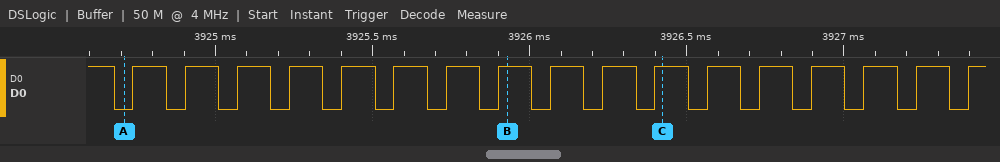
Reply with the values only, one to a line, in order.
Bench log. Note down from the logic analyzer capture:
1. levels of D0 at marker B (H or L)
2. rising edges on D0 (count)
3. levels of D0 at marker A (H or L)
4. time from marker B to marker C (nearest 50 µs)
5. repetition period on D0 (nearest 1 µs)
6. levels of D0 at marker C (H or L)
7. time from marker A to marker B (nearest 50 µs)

D0=H
17
D0=L
500 µs
166 µs
D0=H
1200 µs
